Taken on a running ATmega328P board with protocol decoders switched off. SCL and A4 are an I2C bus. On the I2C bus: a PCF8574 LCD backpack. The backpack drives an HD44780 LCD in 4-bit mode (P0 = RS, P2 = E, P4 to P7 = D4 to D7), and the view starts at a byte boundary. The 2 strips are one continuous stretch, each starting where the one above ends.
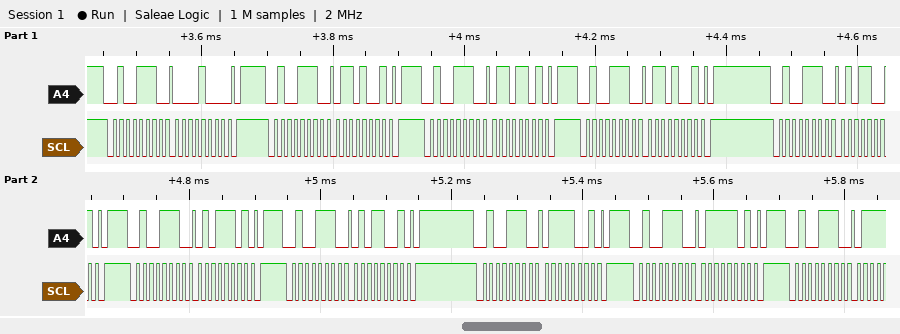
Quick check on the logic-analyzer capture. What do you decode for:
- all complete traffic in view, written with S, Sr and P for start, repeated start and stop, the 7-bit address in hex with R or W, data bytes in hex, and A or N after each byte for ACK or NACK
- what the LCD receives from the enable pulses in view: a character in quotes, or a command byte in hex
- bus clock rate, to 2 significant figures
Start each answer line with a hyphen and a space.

- S 27W A 08 A P S 27W A 69 A P S 27W A 6D A P S 27W A 69 A P S 27W A 59 A P S 27W A 5D A P S 27W A 59 A P S 27W A 79 A P S 27W A 7D A P S 27W A
- 'e'
- 100 kHz
